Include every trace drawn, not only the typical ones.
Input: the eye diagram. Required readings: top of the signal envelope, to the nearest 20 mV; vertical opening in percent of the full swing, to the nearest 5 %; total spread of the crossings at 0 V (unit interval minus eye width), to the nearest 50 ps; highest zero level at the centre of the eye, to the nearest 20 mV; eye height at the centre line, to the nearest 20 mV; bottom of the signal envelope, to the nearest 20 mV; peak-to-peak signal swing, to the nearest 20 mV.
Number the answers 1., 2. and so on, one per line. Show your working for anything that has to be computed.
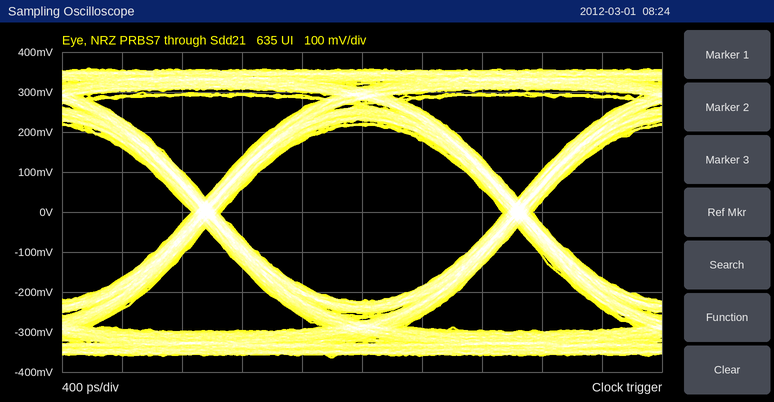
1. 360 mV
2. 440 mV / 720 mV ≈ 61.1 %, so 60 % to the nearest 5 %
3. 200 ps
4. -220 mV
5. 440 mV
6. -360 mV
7. 720 mV
